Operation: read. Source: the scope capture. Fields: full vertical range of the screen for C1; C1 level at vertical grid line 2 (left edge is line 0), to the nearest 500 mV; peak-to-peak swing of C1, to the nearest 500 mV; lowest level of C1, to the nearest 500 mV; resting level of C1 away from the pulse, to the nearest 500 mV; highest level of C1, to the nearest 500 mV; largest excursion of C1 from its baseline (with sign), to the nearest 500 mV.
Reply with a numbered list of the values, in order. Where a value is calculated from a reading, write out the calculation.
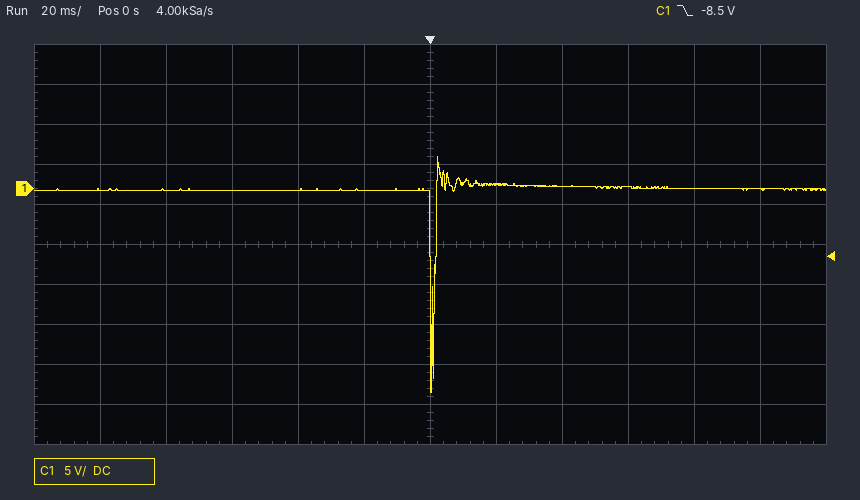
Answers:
1. 50 V
2. 0.0 V
3. 4.0 V − (-25.5 V) = 29.5 V
4. -25.5 V
5. 0.0 V
6. 4.0 V
7. -25.5 V − (0.0 V) = -25.5 V
